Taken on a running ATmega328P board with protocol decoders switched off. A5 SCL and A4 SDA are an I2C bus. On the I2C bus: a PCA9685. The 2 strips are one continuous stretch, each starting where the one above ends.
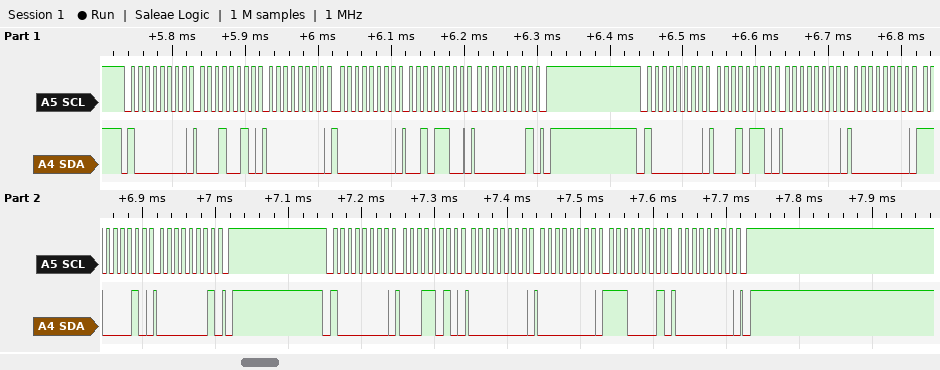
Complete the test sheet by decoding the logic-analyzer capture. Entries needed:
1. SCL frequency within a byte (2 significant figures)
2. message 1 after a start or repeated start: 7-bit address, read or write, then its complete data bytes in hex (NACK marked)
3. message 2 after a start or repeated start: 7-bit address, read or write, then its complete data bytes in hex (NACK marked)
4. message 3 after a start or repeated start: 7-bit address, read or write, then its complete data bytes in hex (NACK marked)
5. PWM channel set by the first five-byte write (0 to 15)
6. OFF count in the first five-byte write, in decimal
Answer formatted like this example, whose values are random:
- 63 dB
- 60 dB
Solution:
- 100 kHz
- 0x40 write: 12 00 00 2C 01
- 0x40 write: 16 00 00 C2 01
- 0x40 write: 1A 00 00 E1 00
- 3
- 300
